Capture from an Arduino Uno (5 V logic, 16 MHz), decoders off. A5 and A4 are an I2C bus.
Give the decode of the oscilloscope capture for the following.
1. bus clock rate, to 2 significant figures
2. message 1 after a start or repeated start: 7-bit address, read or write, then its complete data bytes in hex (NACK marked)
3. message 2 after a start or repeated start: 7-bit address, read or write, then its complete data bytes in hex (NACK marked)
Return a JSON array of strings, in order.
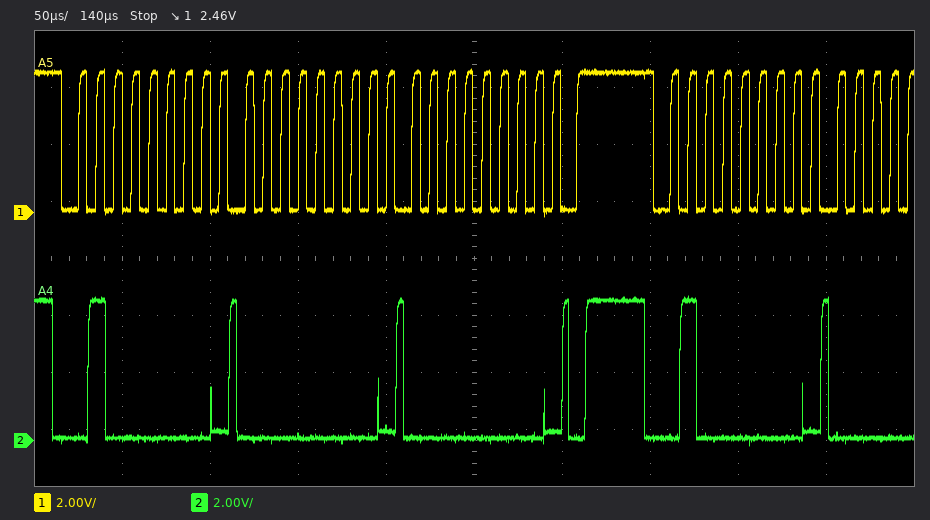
["100 kHz", "0x20 write: 00 00", "0x20 write"]
